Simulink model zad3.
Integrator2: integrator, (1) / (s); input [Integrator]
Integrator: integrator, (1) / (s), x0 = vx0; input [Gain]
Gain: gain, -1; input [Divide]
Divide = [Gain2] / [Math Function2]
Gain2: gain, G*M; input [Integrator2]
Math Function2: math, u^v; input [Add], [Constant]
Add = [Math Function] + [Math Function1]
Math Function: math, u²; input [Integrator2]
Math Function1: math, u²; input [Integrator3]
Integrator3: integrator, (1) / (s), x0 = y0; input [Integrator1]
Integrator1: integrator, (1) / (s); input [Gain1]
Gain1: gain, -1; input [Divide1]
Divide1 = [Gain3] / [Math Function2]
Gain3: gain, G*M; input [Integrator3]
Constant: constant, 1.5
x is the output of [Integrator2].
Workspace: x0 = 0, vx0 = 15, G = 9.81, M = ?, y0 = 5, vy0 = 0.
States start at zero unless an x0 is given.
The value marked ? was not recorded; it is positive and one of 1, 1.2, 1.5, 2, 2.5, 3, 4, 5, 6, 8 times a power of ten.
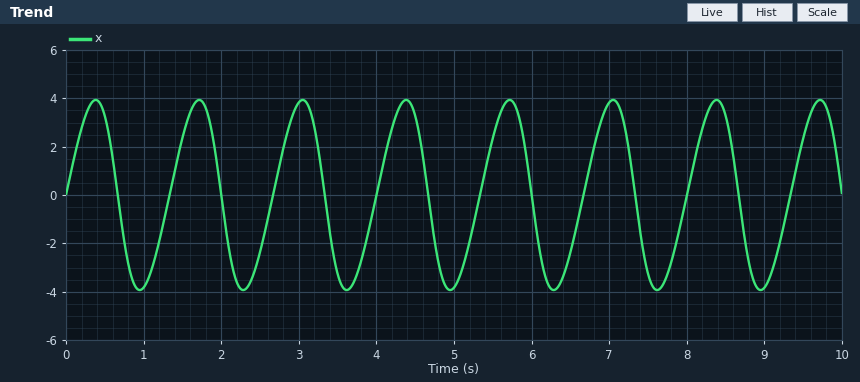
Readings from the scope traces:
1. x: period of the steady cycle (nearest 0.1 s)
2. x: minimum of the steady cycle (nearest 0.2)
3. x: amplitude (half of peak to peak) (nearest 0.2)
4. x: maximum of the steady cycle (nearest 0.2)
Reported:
1.3 s
-4.0
4.0
4.0
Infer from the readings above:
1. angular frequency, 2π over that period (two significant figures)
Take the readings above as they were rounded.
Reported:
4.8 rad/s
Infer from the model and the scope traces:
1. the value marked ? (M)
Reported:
150
